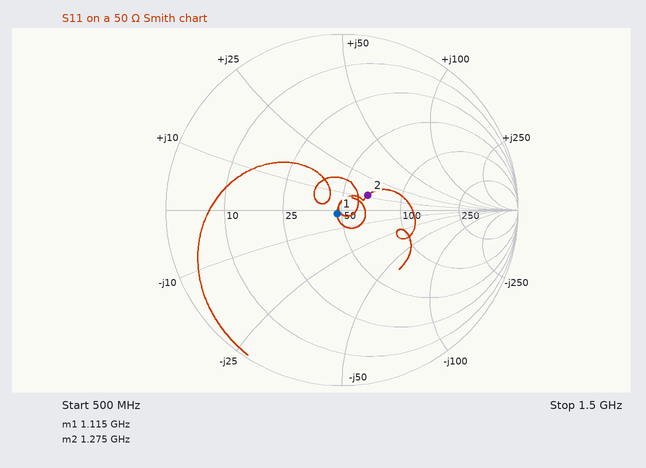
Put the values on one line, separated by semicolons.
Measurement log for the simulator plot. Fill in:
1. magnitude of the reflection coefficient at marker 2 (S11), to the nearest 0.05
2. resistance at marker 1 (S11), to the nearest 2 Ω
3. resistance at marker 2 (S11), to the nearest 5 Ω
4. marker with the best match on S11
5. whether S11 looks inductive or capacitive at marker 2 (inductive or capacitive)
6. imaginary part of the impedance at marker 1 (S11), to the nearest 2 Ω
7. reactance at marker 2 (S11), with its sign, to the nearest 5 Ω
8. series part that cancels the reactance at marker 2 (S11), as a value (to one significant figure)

0.15; 48 Ω; 65 Ω; marker 1; inductive; -2 Ω; +10 Ω; 10 pF
